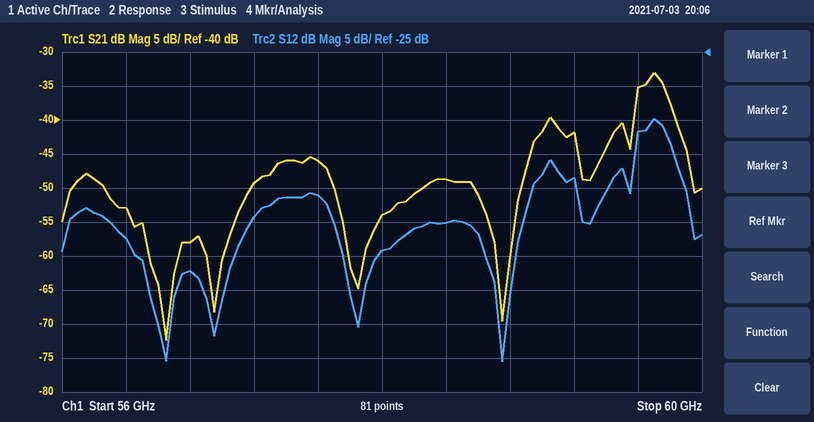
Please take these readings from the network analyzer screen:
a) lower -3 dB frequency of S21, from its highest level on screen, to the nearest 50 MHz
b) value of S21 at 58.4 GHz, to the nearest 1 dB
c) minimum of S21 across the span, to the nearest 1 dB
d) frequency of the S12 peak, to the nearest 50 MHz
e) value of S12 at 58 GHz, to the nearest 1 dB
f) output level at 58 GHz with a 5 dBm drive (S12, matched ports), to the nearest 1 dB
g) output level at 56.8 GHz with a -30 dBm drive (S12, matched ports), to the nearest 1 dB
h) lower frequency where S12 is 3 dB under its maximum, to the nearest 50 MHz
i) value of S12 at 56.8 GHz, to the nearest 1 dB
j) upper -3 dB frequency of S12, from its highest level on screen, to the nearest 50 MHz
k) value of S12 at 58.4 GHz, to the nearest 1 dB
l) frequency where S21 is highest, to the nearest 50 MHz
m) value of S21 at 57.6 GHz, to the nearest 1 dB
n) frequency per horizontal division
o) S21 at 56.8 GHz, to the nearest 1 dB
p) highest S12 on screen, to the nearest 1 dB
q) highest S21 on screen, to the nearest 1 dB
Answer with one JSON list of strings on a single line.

["59.60 GHz", "-49 dB", "-72 dB", "59.70 GHz", "-54 dB", "-49 dBm", "-87 dBm", "59.60 GHz", "-57 dB", "59.80 GHz", "-50 dB", "59.70 GHz", "-46 dB", "400 MHz", "-58 dB", "-35 dB", "-33 dB"]
